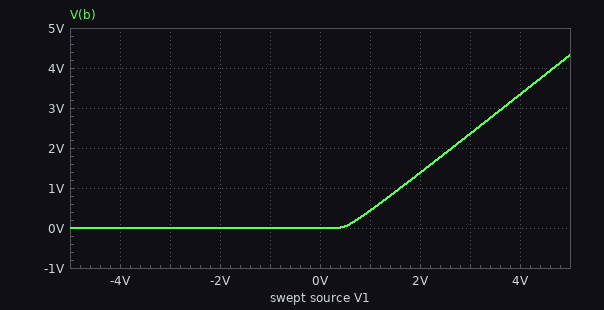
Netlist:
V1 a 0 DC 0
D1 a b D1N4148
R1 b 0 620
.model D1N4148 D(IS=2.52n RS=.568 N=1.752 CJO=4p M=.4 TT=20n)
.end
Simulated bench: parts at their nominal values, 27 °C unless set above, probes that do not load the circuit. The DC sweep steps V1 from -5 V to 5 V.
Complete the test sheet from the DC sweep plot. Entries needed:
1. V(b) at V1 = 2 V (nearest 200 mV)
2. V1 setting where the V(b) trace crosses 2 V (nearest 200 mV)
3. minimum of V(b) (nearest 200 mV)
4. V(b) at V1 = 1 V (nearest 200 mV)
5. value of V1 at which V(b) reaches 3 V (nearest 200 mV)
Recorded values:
1.4 V
2.6 V
0 V
400 mV
3.6 V
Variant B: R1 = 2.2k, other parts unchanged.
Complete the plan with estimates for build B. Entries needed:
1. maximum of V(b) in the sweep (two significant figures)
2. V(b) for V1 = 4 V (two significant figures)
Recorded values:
4.4 V
3.4 V
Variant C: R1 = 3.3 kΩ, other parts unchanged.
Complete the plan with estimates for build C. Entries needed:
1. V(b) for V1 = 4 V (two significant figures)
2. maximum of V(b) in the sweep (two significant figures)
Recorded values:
3.4 V
4.4 V
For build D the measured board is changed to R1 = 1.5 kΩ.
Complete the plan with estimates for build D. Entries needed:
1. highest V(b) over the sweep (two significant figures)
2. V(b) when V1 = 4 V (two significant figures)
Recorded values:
4.4 V
3.4 V
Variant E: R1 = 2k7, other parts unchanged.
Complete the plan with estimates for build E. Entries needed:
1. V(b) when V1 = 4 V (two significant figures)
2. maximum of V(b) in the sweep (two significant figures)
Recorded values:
3.4 V
4.4 V
